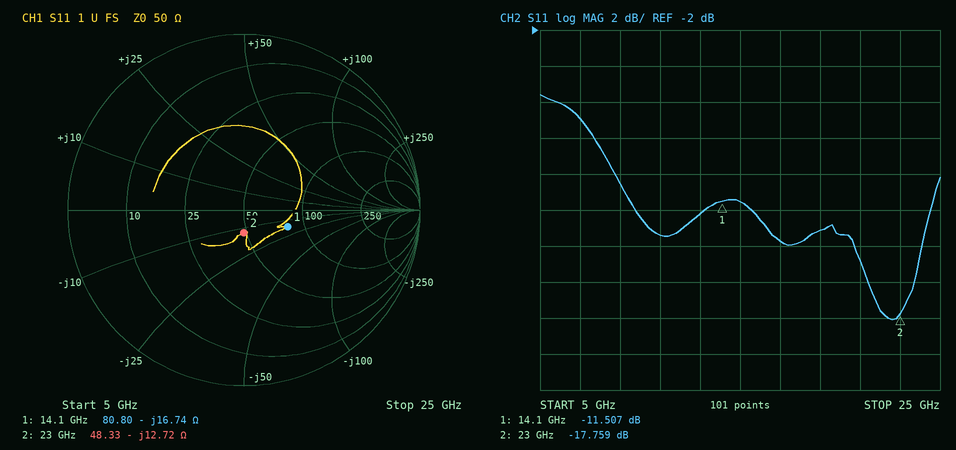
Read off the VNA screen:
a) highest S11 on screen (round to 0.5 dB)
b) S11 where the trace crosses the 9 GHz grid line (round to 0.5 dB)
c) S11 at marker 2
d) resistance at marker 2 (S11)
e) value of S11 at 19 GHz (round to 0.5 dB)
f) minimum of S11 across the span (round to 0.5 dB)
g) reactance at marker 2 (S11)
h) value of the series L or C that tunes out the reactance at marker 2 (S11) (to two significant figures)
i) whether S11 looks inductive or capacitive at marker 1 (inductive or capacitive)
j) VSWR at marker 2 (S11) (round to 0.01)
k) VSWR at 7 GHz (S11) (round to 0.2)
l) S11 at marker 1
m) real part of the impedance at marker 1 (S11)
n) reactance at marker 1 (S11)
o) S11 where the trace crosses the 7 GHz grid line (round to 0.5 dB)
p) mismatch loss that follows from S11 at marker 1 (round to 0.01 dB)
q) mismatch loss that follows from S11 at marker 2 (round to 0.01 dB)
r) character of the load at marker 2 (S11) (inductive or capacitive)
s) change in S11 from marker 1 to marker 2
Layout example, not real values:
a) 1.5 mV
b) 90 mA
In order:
a) -5.5 dB
b) -10.5 dB
c) -17.759 dB
d) 48.33 Ω
e) -13.0 dB
f) -18.0 dB
g) -12.72 Ω
h) 88 pH
i) capacitive
j) 1.30
k) 2.6
l) -11.507 dB
m) 80.80 Ω
n) -16.74 Ω
o) -7.0 dB
p) 0.32 dB
q) 0.07 dB
r) capacitive
s) -6.252 dB
